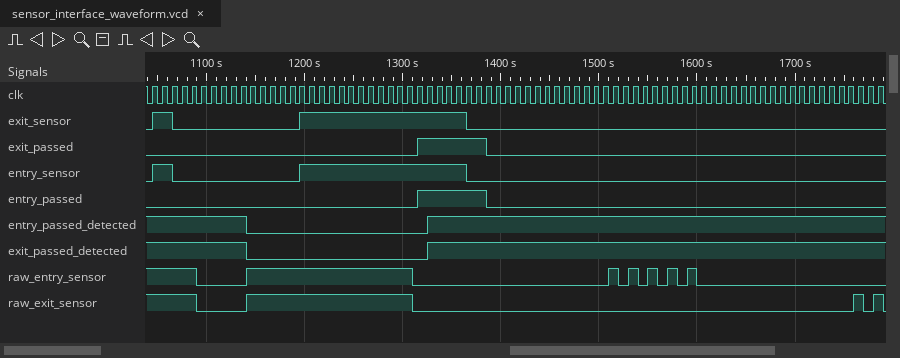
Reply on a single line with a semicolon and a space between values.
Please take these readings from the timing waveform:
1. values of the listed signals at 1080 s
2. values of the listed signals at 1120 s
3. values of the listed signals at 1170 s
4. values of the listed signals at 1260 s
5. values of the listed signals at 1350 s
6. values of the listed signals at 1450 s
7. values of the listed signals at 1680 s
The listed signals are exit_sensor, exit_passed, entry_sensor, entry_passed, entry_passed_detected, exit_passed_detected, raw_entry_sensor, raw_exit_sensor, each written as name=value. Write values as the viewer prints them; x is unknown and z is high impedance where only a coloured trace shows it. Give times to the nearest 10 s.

exit_sensor=0, exit_passed=0, entry_sensor=0, entry_passed=0, entry_passed_detected=1, exit_passed_detected=1, raw_entry_sensor=1, raw_exit_sensor=1; exit_sensor=0, exit_passed=0, entry_sensor=0, entry_passed=0, entry_passed_detected=1, exit_passed_detected=1, raw_entry_sensor=0, raw_exit_sensor=0; exit_sensor=0, exit_passed=0, entry_sensor=0, entry_passed=0, entry_passed_detected=0, exit_passed_detected=0, raw_entry_sensor=1, raw_exit_sensor=1; exit_sensor=1, exit_passed=0, entry_sensor=1, entry_passed=0, entry_passed_detected=0, exit_passed_detected=0, raw_entry_sensor=1, raw_exit_sensor=1; exit_sensor=1, exit_passed=1, entry_sensor=1, entry_passed=1, entry_passed_detected=1, exit_passed_detected=1, raw_entry_sensor=0, raw_exit_sensor=0; exit_sensor=0, exit_passed=0, entry_sensor=0, entry_passed=0, entry_passed_detected=1, exit_passed_detected=1, raw_entry_sensor=0, raw_exit_sensor=0; exit_sensor=0, exit_passed=0, entry_sensor=0, entry_passed=0, entry_passed_detected=1, exit_passed_detected=1, raw_entry_sensor=0, raw_exit_sensor=0
